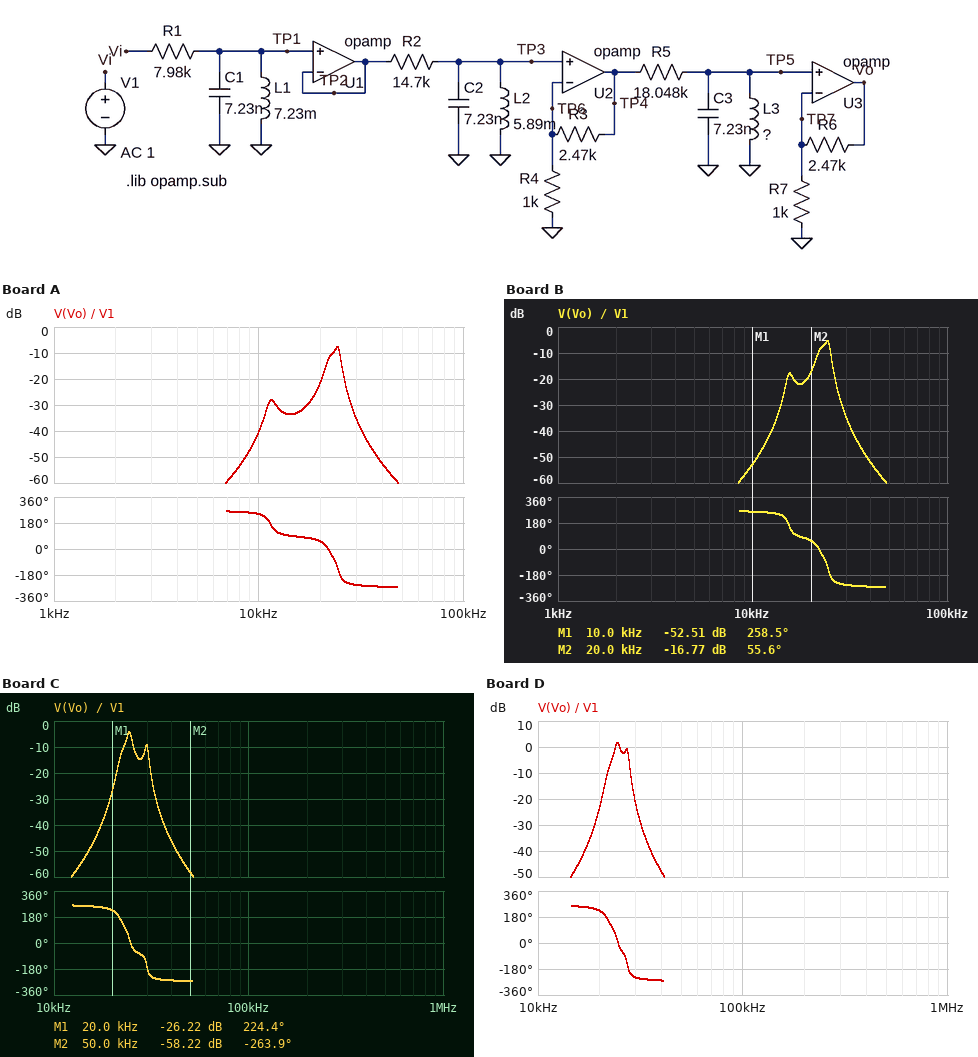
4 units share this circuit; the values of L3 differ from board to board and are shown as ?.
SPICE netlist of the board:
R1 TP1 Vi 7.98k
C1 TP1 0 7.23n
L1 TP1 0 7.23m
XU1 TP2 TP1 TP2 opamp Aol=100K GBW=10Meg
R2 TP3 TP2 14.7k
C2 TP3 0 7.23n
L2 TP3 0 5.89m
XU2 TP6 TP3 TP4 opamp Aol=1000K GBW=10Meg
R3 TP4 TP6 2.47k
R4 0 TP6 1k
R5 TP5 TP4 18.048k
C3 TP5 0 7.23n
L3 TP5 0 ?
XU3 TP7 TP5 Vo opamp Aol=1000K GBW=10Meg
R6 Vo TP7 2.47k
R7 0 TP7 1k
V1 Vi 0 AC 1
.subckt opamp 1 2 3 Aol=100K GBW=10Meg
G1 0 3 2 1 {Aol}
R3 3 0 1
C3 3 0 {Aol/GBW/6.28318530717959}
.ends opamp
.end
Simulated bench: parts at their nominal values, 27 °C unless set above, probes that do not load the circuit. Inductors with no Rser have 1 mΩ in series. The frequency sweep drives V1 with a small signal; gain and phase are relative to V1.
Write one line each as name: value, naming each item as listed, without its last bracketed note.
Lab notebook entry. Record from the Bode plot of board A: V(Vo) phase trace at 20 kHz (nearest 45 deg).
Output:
V(Vo) phase trace at 20 kHz: 45 deg
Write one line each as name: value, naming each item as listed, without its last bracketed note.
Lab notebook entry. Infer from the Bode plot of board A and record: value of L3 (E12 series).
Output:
value of L3: 27 mH
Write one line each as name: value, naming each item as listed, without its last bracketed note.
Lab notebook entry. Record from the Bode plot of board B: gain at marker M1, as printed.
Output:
gain at marker M1, as printed: -52.51 dB
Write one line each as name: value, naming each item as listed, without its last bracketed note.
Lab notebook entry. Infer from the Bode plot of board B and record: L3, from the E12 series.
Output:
L3, from the E12 series: 15 mH
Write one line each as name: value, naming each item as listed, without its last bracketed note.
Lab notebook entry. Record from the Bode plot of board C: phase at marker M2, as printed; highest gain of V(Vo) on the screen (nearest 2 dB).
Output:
phase at marker M2, as printed: -263.9 deg
highest gain of V(Vo) on the screen: -4 dB
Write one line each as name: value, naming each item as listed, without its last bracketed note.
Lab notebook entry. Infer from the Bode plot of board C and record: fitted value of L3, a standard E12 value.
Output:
fitted value of L3, a standard E12 value: 3.9 mH
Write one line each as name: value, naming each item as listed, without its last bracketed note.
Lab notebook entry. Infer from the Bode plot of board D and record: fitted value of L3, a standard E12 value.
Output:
fitted value of L3, a standard E12 value: 4.7 mH
